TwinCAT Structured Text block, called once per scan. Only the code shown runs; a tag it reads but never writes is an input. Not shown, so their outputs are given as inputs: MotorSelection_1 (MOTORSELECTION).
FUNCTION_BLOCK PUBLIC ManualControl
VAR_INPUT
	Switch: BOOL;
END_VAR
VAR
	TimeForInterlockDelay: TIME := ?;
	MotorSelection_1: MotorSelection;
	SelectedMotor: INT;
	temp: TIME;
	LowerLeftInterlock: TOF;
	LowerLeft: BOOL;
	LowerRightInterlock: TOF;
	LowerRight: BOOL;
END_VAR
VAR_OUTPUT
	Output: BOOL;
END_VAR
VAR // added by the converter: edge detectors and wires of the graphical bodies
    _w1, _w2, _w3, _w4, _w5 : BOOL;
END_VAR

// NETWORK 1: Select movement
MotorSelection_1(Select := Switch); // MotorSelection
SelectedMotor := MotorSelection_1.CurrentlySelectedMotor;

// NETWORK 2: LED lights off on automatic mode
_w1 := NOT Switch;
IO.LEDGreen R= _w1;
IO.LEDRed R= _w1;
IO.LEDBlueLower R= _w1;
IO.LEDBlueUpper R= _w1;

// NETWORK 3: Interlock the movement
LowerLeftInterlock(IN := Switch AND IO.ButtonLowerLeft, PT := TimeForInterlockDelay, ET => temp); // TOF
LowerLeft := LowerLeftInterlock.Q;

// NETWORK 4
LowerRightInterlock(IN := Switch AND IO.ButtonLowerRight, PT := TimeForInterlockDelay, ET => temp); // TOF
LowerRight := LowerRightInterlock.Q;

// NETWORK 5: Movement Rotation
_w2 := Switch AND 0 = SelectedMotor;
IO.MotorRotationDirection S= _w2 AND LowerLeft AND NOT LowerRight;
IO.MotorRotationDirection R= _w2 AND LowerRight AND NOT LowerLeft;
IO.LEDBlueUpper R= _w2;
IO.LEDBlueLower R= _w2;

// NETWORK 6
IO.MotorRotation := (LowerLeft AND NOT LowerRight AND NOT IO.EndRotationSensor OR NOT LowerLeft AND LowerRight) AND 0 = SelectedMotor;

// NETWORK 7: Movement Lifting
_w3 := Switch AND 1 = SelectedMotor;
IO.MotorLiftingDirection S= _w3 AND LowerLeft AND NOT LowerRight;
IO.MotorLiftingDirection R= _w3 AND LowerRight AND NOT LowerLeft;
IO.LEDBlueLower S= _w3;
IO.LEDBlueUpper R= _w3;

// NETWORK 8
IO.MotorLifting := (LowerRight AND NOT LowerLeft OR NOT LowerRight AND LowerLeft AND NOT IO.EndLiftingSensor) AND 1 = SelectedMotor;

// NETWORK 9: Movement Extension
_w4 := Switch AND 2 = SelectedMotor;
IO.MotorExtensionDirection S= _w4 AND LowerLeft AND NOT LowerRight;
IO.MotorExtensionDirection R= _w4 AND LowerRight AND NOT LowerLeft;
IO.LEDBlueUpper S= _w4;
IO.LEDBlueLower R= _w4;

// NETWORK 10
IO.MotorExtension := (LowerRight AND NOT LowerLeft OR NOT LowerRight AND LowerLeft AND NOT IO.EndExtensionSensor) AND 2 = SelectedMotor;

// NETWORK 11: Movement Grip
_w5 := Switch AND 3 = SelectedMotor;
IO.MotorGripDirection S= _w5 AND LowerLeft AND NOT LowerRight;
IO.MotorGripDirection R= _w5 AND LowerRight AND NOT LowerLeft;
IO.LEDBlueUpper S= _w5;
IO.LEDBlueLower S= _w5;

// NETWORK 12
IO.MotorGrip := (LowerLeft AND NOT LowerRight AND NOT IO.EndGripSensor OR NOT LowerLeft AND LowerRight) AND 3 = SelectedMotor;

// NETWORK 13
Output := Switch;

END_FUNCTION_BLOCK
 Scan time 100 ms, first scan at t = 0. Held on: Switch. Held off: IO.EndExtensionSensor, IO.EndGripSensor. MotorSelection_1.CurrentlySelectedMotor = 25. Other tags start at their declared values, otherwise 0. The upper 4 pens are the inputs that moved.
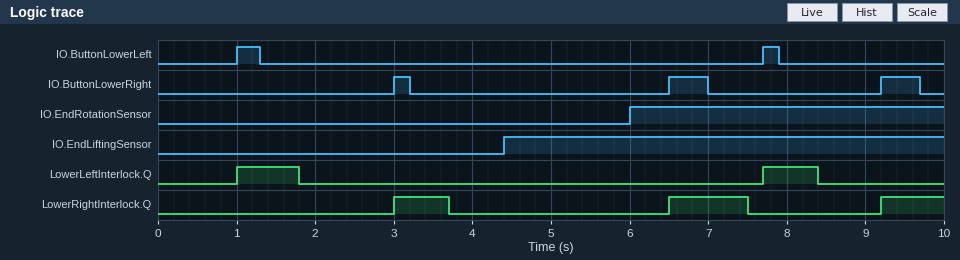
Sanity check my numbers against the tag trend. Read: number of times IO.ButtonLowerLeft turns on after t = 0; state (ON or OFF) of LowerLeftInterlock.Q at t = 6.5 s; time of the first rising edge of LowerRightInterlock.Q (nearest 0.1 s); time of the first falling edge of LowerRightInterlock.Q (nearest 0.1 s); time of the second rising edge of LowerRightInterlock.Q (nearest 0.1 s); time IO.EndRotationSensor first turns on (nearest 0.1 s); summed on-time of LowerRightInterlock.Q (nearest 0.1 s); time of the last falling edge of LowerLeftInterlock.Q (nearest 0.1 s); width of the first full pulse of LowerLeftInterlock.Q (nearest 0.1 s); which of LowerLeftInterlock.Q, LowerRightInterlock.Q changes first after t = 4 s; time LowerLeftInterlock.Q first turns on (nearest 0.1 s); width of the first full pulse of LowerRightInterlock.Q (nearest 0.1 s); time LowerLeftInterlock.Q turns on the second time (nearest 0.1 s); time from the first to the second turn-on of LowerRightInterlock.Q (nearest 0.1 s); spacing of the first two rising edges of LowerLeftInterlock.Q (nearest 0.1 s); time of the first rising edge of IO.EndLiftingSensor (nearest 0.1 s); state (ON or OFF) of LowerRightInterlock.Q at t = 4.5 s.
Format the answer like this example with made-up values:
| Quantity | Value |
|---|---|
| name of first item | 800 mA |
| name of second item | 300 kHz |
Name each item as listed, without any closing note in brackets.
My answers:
| Quantity | Value |
|---|---|
| number of times IO.ButtonLowerLeft turns on after t = 0 | 2 |
| state (ON or OFF) of LowerLeftInterlock.Q at t = 6.5 s | OFF |
| time of the first rising edge of LowerRightInterlock.Q | 3.0 s |
| time of the first falling edge of LowerRightInterlock.Q | 3.7 s |
| time of the second rising edge of LowerRightInterlock.Q | 6.5 s |
| time IO.EndRotationSensor first turns on | 6.0 s |
| summed on-time of LowerRightInterlock.Q | 2.5 s |
| time of the last falling edge of LowerLeftInterlock.Q | 8.4 s |
| width of the first full pulse of LowerLeftInterlock.Q | 0.8 s |
| which of LowerLeftInterlock.Q, LowerRightInterlock.Q changes first after t = 4 s | LowerRightInterlock.Q |
| time LowerLeftInterlock.Q first turns on | 1.0 s |
| width of the first full pulse of LowerRightInterlock.Q | 0.7 s |
| time LowerLeftInterlock.Q turns on the second time | 7.7 s |
| time from the first to the second turn-on of LowerRightInterlock.Q | 3.5 s |
| spacing of the first two rising edges of LowerLeftInterlock.Q | 6.7 s |
| time of the first rising edge of IO.EndLiftingSensor | 4.4 s |
| state (ON or OFF) of LowerRightInterlock.Q at t = 4.5 s | OFF |
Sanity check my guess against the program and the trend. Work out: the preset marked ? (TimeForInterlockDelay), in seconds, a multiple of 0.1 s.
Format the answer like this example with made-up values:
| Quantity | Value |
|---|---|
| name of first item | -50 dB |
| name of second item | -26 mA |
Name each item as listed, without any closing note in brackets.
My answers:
| Quantity | Value |
|---|---|
| the preset marked ? (TimeForInterlockDelay), in seconds, a multiple of 0.1 s | 0.5 s |
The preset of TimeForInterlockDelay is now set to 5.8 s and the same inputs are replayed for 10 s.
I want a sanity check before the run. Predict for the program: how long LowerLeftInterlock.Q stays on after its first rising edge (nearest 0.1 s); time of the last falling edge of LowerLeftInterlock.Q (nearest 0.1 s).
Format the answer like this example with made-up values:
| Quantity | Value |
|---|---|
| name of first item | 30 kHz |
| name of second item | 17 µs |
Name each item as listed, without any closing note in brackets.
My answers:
| Quantity | Value |
|---|---|
| how long LowerLeftInterlock.Q stays on after its first rising edge | 6.1 s |
| time of the last falling edge of LowerLeftInterlock.Q | 7.1 s |
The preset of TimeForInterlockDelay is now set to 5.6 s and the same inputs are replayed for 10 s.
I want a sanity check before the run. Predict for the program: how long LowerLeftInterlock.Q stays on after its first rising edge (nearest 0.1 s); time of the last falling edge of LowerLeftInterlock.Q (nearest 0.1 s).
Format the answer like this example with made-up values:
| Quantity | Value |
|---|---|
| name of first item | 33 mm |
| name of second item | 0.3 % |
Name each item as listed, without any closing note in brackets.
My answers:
| Quantity | Value |
|---|---|
| how long LowerLeftInterlock.Q stays on after its first rising edge | 5.9 s |
| time of the last falling edge of LowerLeftInterlock.Q | 6.9 s |
